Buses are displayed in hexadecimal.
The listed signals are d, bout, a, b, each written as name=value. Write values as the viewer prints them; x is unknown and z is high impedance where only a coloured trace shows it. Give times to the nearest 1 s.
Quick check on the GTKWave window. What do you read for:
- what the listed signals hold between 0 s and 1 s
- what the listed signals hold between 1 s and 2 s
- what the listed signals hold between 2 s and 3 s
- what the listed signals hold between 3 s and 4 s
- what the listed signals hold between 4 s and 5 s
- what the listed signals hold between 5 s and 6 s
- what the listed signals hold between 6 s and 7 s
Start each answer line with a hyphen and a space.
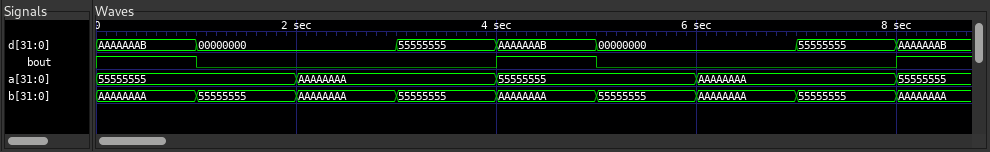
- d=AAAAAAAB, bout=1, a=55555555, b=AAAAAAAA
- d=00000000, bout=0, a=55555555, b=55555555
- d=00000000, bout=0, a=AAAAAAAA, b=AAAAAAAA
- d=55555555, bout=0, a=AAAAAAAA, b=55555555
- d=AAAAAAAB, bout=1, a=55555555, b=AAAAAAAA
- d=00000000, bout=0, a=55555555, b=55555555
- d=00000000, bout=0, a=AAAAAAAA, b=AAAAAAAA
